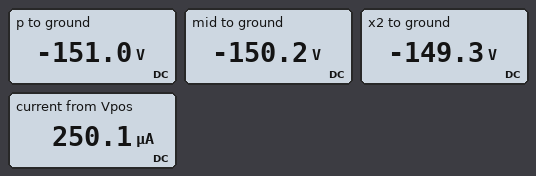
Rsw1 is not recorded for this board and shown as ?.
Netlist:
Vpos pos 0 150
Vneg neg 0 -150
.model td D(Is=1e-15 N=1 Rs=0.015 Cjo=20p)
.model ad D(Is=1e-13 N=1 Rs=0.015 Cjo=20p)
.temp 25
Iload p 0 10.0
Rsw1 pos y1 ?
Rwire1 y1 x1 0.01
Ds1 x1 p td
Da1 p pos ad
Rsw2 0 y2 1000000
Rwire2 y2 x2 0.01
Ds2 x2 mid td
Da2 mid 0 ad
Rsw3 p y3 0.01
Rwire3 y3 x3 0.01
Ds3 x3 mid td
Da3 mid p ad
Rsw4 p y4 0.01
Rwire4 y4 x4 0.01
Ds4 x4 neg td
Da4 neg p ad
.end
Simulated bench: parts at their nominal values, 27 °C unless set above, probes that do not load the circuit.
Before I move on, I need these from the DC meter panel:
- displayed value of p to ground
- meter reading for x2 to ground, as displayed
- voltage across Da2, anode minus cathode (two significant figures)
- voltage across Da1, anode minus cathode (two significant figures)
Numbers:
-151.0 V
-149.3 V
-150 V
-300 V
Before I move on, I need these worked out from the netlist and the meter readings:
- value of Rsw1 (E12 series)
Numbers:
1.2 MΩ
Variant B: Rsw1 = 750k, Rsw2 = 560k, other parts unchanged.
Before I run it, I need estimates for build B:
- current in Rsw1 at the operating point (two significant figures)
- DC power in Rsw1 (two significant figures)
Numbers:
400 µA
120 mW
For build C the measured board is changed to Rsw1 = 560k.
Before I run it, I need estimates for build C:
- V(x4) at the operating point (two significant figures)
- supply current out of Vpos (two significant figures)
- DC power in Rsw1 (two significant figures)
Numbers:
-150 V
540 µA
160 mW
